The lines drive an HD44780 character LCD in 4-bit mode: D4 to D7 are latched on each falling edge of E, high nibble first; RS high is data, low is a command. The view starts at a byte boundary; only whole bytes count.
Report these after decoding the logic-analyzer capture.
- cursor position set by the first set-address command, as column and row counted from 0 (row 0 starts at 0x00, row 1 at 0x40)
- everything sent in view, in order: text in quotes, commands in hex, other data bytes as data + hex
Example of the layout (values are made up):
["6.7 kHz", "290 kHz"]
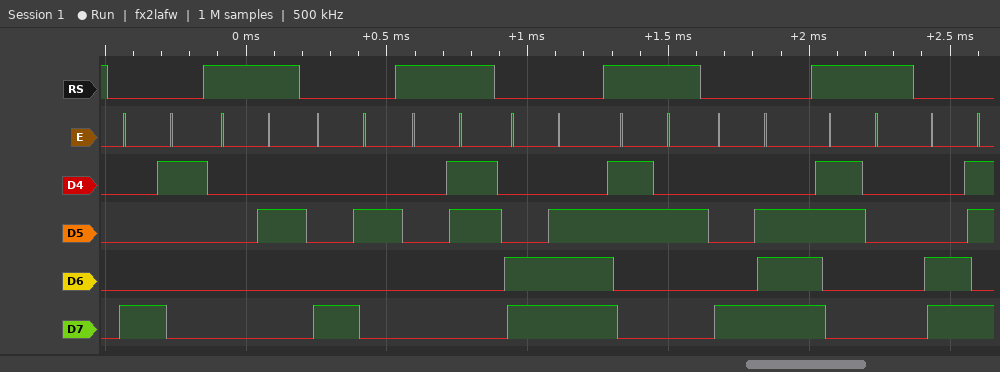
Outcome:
["column 1, row 0", "0x81 data 02 0x82 data 03 0xCE \"2\" 0x8E \"0\" 0xCB"]
